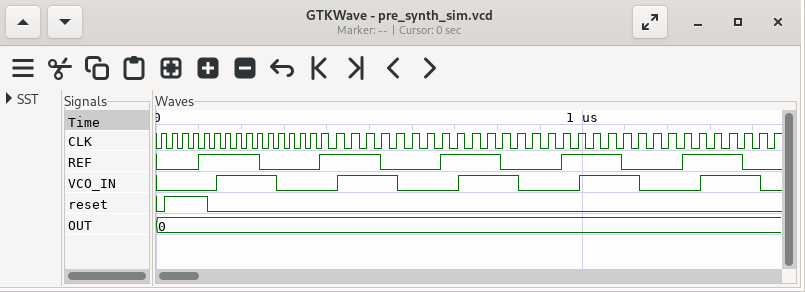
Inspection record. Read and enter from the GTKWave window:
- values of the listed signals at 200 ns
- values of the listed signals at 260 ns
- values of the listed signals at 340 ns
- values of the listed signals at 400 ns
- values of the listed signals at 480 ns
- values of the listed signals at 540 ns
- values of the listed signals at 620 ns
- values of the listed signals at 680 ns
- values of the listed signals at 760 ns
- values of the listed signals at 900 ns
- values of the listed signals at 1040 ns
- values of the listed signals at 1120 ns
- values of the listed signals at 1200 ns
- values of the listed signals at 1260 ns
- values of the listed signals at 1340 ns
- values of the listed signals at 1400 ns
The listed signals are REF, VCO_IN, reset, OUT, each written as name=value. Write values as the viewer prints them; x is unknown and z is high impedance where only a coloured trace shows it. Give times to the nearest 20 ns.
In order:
REF=1, VCO_IN=1, reset=0, OUT=0
REF=0, VCO_IN=1, reset=0, OUT=0
REF=0, VCO_IN=0, reset=0, OUT=0
REF=1, VCO_IN=0, reset=0, OUT=0
REF=1, VCO_IN=1, reset=0, OUT=0
REF=0, VCO_IN=1, reset=0, OUT=0
REF=0, VCO_IN=0, reset=0, OUT=0
REF=1, VCO_IN=0, reset=0, OUT=0
REF=1, VCO_IN=1, reset=0, OUT=0
REF=0, VCO_IN=0, reset=0, OUT=0
REF=1, VCO_IN=1, reset=0, OUT=0
REF=0, VCO_IN=1, reset=0, OUT=0
REF=0, VCO_IN=0, reset=0, OUT=0
REF=1, VCO_IN=0, reset=0, OUT=0
REF=1, VCO_IN=1, reset=0, OUT=0
REF=0, VCO_IN=1, reset=0, OUT=0
